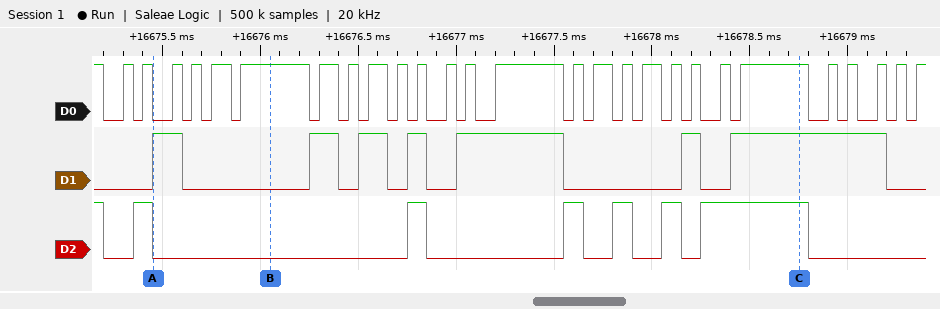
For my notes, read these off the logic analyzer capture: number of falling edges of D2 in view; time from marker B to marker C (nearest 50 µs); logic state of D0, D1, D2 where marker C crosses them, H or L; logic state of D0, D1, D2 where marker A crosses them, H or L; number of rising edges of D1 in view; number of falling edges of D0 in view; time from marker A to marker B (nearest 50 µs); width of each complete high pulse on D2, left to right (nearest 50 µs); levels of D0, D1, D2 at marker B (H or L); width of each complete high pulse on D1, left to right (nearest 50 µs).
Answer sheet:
7
2700 µs
D0=H, D1=H, D2=H
D0=L, D1=H, D2=L
7
27
600 µs
100 µs, 100 µs, 100 µs, 100 µs, 100 µs, 550 µs
D0=H, D1=L, D2=L
150 µs, 150 µs, 150 µs, 100 µs, 550 µs, 100 µs, 800 µs
